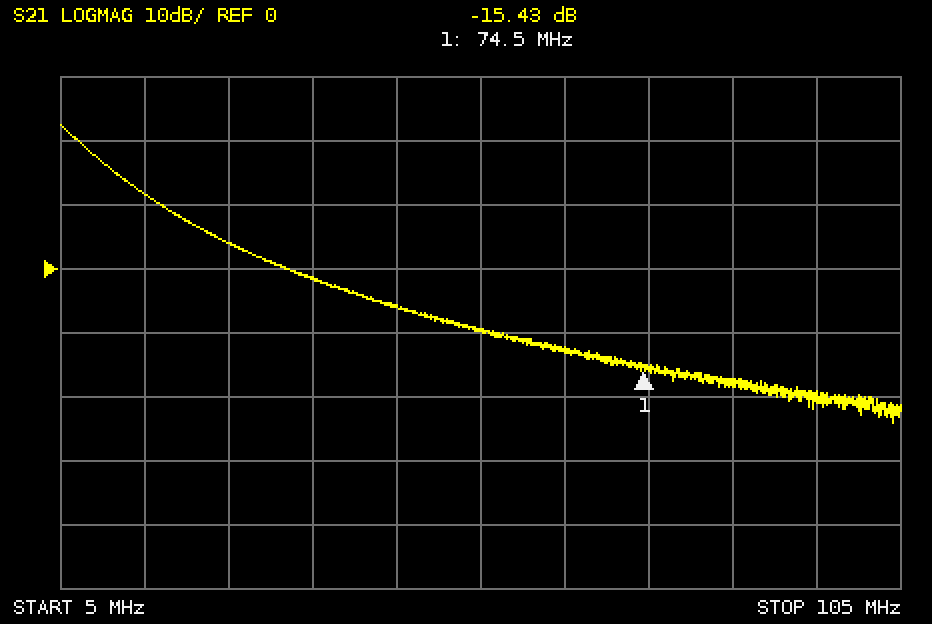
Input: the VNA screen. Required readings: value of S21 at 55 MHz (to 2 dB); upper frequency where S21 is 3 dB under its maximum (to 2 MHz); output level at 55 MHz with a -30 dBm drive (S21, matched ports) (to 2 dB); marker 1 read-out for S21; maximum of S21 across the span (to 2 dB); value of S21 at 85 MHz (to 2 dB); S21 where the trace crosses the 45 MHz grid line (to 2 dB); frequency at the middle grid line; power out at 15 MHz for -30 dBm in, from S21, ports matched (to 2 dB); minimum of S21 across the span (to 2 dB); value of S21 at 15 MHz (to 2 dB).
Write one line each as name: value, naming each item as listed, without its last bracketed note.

value of S21 at 55 MHz: -10 dB
upper frequency where S21 is 3 dB under its maximum: 8 MHz
output level at 55 MHz with a -30 dBm drive (S21, matched ports): -40 dBm
marker 1 read-out for S21: -15.43 dB
maximum of S21 across the span: 22 dB
value of S21 at 85 MHz: -18 dB
S21 where the trace crosses the 45 MHz grid line: -6 dB
frequency at the middle grid line: 55 MHz
power out at 15 MHz for -30 dBm in, from S21, ports matched: -18 dBm
minimum of S21 across the span: -24 dB
value of S21 at 15 MHz: 12 dB
